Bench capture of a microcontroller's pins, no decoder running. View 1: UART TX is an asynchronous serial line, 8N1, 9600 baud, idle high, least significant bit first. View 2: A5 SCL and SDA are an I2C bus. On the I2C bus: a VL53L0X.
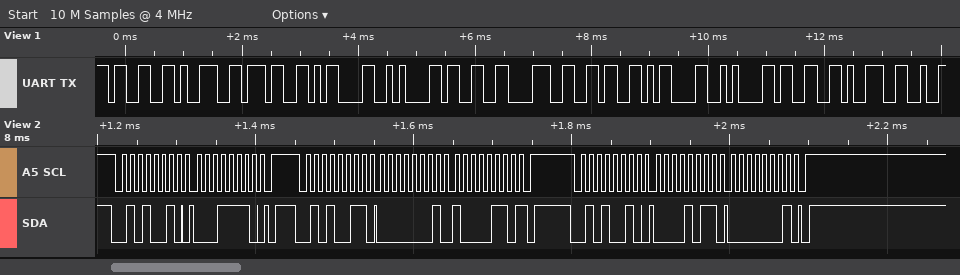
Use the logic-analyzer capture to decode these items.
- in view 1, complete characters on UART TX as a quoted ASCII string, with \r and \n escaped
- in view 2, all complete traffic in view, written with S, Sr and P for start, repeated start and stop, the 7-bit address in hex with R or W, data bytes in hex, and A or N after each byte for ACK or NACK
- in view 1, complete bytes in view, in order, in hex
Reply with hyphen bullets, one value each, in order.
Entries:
- "397\r\n386\r\n39"
- S 29W A 1E A P S 29R A 01 A 86 N P S 29W A 0B A 01 A P
- 33 39 37 0D 0A 33 38 36 0D 0A 33 39
